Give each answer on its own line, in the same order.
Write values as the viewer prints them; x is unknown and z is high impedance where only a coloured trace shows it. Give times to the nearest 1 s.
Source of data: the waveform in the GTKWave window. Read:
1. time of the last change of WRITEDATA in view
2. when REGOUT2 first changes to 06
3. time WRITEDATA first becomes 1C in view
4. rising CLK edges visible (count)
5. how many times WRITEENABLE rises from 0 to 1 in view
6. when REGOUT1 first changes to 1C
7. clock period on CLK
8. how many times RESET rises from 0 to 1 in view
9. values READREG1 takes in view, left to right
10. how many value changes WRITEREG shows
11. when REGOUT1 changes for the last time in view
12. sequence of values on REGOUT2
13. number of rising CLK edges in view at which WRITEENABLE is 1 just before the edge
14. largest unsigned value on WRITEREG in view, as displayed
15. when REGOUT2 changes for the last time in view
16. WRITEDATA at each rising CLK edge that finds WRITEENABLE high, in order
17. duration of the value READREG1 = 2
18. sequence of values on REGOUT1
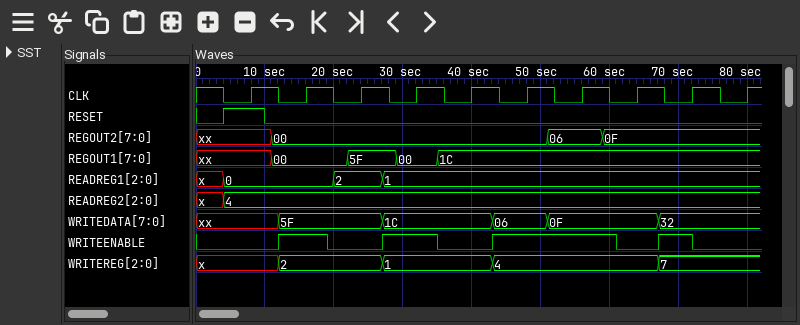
67 s
51 s
27 s
10
4
35 s
8 s
1
x, 0, 2, 1
4
35 s
xx, 00, 06, 0F
5
7
59 s
5F, 1C, 06, 0F, 32
7 s
xx, 00, 5F, 00, 1C
